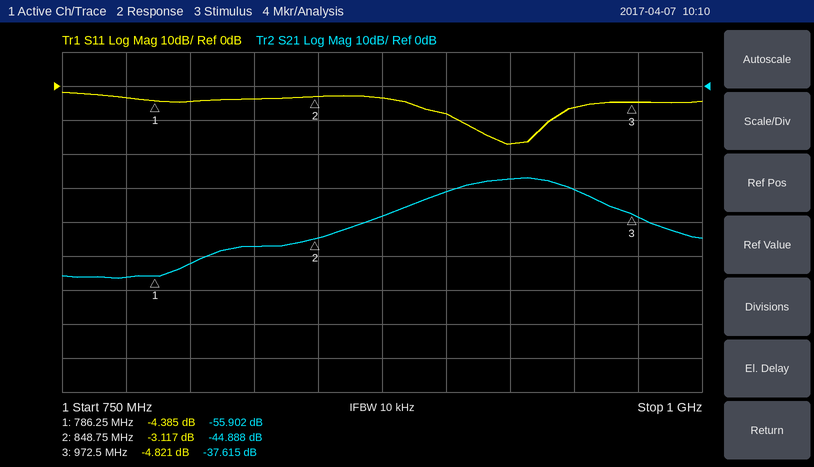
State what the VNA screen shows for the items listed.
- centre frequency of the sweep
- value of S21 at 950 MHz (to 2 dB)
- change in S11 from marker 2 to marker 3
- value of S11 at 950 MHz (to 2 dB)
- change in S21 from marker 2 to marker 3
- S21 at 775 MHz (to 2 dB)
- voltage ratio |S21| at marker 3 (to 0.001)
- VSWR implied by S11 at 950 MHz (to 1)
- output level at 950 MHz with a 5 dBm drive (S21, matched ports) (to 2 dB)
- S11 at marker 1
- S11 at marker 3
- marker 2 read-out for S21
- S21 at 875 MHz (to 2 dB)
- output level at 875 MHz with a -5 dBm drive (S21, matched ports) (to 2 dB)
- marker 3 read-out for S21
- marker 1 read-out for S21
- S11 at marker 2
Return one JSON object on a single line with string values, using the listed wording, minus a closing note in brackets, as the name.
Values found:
{"centre frequency of the sweep": "875 MHz", "value of S21 at 950 MHz": "-30 dB", "change in S11 from marker 2 to marker 3": "-1.704 dB", "value of S11 at 950 MHz": "-6 dB", "change in S21 from marker 2 to marker 3": "7.273 dB", "S21 at 775 MHz": "-56 dB", "voltage ratio |S21| at marker 3": "0.013", "VSWR implied by S11 at 950 MHz": "3", "output level at 950 MHz with a 5 dBm drive (S21, matched ports)": "-26 dBm", "S11 at marker 1": "-4.385 dB", "S11 at marker 3": "-4.821 dB", "marker 2 read-out for S21": "-44.888 dB", "S21 at 875 MHz": "-38 dB", "output level at 875 MHz with a -5 dBm drive (S21, matched ports)": "-44 dBm", "marker 3 read-out for S21": "-37.615 dB", "marker 1 read-out for S21": "-55.902 dB", "S11 at marker 2": "-3.117 dB"}
